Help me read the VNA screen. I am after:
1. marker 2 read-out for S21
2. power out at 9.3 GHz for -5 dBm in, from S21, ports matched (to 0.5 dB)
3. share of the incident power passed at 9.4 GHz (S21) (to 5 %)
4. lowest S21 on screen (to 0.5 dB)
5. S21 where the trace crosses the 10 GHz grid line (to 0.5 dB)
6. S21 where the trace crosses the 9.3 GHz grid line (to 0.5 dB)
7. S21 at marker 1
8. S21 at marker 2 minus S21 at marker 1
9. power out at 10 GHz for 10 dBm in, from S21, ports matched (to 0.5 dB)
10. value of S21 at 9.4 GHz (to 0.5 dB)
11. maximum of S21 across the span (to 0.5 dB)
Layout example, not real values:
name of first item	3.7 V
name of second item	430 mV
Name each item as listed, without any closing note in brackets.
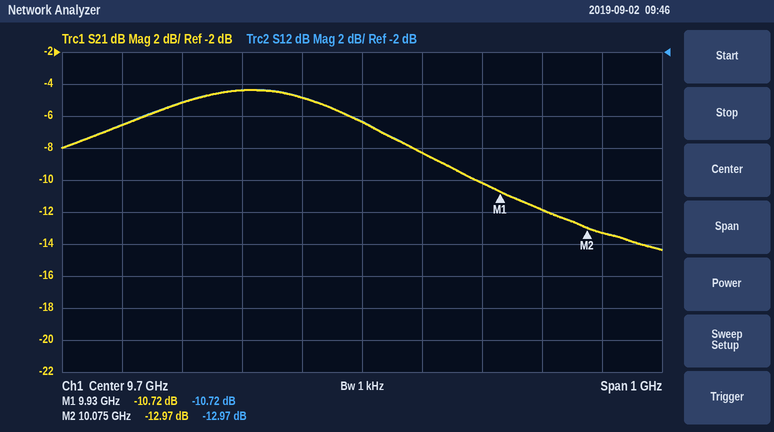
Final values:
marker 2 read-out for S21	-12.97 dB
power out at 9.3 GHz for -5 dBm in, from S21, ports matched	-11.5 dBm
share of the incident power passed at 9.4 GHz (S21)	30 %
lowest S21 on screen	-14.5 dB
S21 where the trace crosses the 10 GHz grid line	-12.0 dB
S21 where the trace crosses the 9.3 GHz grid line	-6.5 dB
S21 at marker 1	-10.72 dB
S21 at marker 2 minus S21 at marker 1	-2.25 dB
power out at 10 GHz for 10 dBm in, from S21, ports matched	-2.0 dBm
value of S21 at 9.4 GHz	-5.0 dB
maximum of S21 across the span	-4.5 dB
